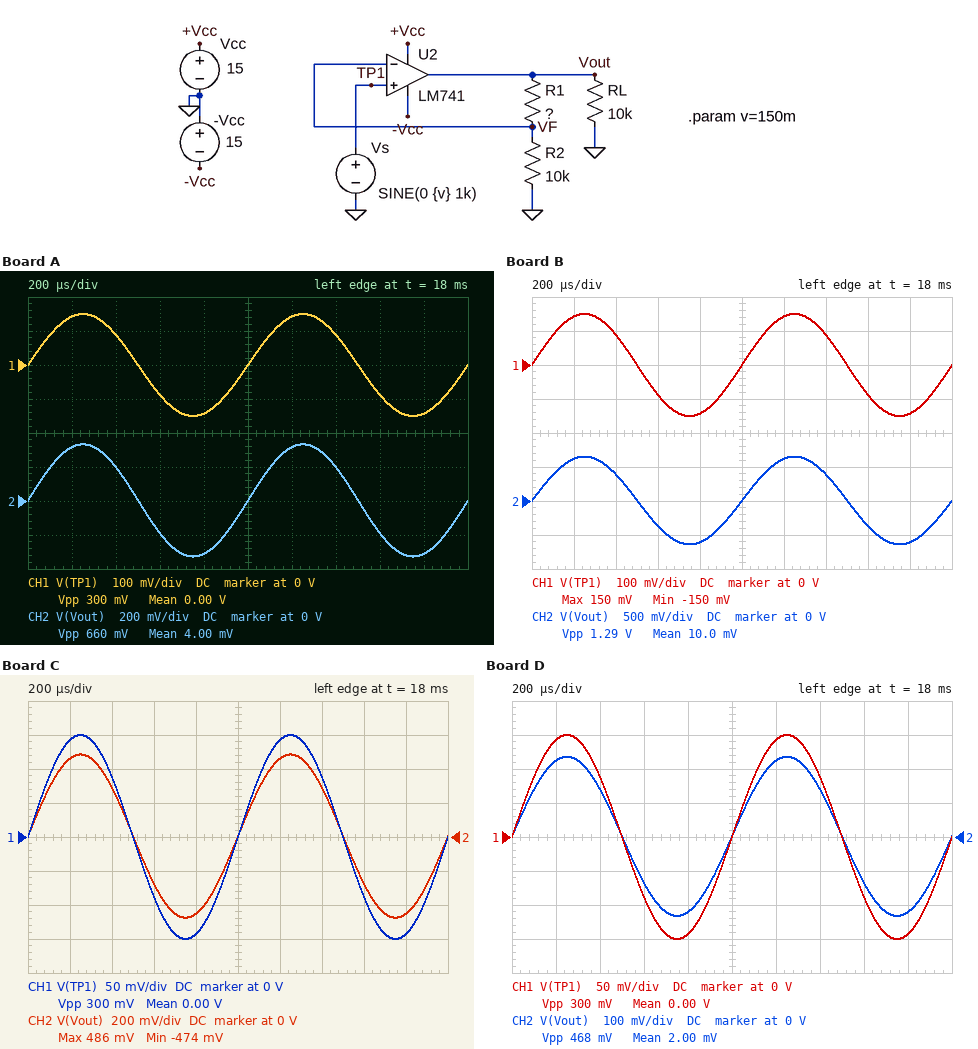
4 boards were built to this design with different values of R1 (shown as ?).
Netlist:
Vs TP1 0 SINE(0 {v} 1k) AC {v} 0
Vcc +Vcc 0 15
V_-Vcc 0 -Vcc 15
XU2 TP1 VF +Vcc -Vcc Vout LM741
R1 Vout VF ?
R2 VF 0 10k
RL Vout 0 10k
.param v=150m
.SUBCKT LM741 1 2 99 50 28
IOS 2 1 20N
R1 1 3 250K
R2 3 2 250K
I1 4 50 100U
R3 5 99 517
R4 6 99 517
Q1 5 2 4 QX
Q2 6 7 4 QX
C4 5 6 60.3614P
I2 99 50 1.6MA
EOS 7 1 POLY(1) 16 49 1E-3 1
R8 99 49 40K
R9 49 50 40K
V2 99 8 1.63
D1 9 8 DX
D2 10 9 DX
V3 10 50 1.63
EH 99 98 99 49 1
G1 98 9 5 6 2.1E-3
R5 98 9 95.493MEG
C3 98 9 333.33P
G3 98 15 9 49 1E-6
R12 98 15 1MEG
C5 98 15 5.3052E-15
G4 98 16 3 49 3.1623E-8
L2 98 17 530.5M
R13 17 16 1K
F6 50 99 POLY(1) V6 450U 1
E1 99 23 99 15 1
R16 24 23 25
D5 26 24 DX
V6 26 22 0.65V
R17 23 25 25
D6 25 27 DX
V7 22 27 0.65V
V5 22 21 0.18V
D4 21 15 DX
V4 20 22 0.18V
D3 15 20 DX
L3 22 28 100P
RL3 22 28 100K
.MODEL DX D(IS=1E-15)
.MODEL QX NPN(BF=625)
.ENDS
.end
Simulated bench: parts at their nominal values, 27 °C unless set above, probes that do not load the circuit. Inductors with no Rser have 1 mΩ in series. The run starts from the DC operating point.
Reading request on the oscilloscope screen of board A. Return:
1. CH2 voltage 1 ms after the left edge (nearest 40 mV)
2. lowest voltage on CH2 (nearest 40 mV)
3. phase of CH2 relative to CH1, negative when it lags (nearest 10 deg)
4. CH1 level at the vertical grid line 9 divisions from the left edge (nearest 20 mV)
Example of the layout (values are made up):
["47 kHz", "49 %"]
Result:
["0 V", "-320 mV", "0 deg", "-140 mV"]
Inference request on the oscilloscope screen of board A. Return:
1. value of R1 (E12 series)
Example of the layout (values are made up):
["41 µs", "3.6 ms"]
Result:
["12 kΩ"]
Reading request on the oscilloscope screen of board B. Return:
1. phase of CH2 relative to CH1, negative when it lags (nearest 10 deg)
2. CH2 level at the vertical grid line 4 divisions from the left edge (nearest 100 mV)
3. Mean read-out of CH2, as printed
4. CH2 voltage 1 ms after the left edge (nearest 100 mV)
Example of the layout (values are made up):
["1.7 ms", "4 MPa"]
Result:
["0 deg", "-600 mV", "10.0 mV", "0 V"]
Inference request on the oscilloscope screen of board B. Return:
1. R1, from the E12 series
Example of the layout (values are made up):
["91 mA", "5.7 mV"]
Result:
["33 kΩ"]
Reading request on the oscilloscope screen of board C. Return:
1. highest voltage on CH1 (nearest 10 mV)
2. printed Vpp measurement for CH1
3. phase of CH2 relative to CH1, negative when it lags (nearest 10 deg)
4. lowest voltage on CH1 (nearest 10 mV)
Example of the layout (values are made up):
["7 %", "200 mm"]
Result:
["150 mV", "300 mV", "0 deg", "-150 mV"]
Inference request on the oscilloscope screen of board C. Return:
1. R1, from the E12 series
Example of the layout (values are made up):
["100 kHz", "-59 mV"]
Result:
["22 kΩ"]
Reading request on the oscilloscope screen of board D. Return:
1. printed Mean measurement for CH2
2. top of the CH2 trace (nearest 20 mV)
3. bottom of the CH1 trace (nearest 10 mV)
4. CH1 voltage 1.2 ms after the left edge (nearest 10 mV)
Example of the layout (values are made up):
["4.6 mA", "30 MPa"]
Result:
["2.00 mV", "240 mV", "-150 mV", "140 mV"]
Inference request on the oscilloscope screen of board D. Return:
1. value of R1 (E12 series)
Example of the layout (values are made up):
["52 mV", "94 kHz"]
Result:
["5.6 kΩ"]
